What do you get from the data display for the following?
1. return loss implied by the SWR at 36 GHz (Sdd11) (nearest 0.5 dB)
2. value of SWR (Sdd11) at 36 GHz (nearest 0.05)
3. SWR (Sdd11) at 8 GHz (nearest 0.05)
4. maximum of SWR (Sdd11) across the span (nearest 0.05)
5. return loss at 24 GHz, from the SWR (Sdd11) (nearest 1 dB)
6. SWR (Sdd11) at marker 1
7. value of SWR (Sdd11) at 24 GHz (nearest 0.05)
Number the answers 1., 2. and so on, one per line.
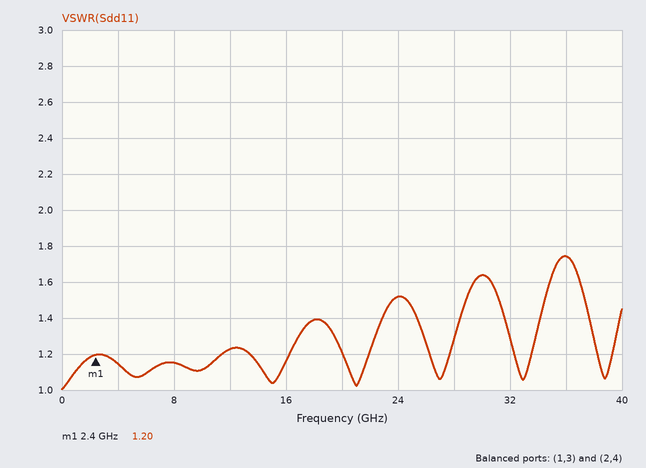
1. 11.5 dB
2. 1.75
3. 1.15
4. 1.75
5. 14 dB
6. 1.20
7. 1.50
